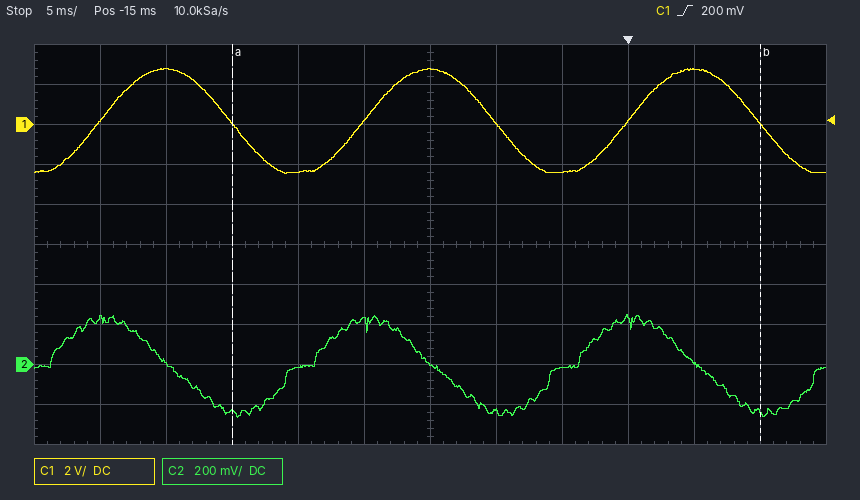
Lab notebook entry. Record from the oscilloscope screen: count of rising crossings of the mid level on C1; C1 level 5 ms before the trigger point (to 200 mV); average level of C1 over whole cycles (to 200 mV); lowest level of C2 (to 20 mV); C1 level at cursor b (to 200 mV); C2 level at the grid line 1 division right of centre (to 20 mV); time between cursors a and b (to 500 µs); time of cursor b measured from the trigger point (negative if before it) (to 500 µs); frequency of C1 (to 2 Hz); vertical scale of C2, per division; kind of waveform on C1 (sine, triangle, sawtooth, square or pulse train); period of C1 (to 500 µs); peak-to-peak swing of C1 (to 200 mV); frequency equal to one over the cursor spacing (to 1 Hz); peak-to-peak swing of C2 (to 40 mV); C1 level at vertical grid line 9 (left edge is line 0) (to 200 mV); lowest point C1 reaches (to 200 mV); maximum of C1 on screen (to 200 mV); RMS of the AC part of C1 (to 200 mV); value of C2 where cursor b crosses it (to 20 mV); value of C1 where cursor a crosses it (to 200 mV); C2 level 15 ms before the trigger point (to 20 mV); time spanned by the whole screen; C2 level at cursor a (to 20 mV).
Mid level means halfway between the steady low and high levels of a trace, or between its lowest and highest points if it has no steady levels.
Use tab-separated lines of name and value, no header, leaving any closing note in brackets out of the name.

count of rising crossings of the mid level on C1	3
C1 level 5 ms before the trigger point	-2.4 V
average level of C1 over whole cycles	200 mV
lowest level of C2	-260 mV
C1 level at cursor b	0.0 V
C2 level at the grid line 1 division right of centre	-240 mV
time between cursors a and b	40.0 ms
time of cursor b measured from the trigger point (negative if before it)	+10.0 ms
frequency of C1	50 Hz
vertical scale of C2, per division	200 mV
kind of waveform on C1	sine
period of C1	20.0 ms
peak-to-peak swing of C1	5.2 V
frequency equal to one over the cursor spacing	25 Hz
peak-to-peak swing of C2	520 mV
C1 level at vertical grid line 9 (left edge is line 0)	200 mV
lowest point C1 reaches	-2.4 V
maximum of C1 on screen	2.8 V
RMS of the AC part of C1	1.8 V
value of C2 where cursor b crosses it	-240 mV
value of C1 where cursor a crosses it	0.0 V
C2 level 15 ms before the trigger point	0 mV
time spanned by the whole screen	60 ms
C2 level at cursor a	-240 mV
